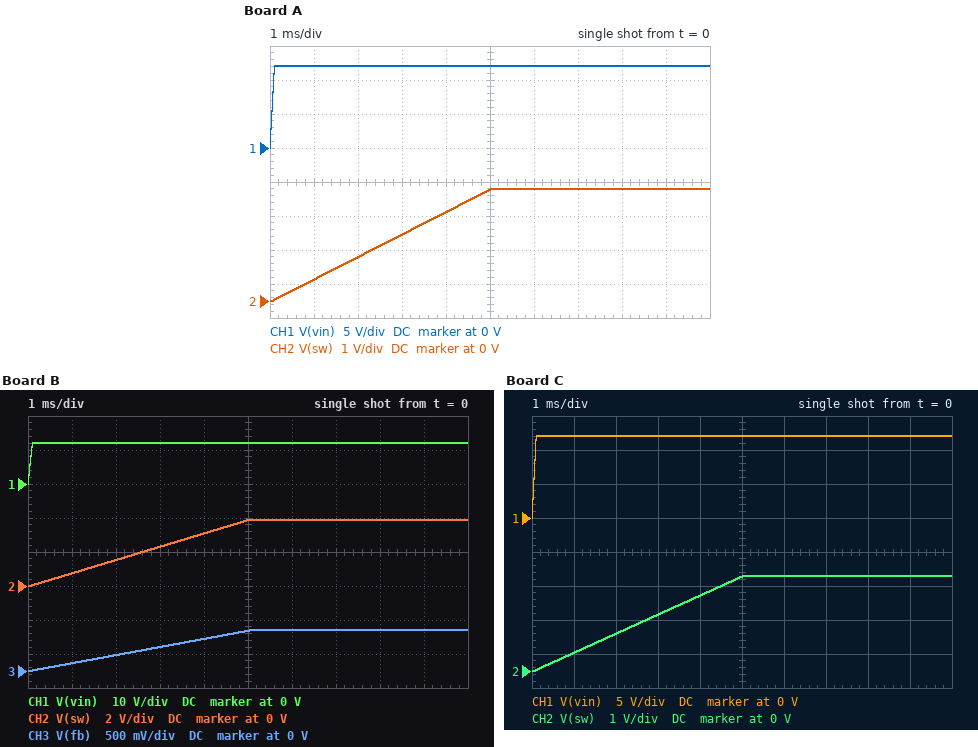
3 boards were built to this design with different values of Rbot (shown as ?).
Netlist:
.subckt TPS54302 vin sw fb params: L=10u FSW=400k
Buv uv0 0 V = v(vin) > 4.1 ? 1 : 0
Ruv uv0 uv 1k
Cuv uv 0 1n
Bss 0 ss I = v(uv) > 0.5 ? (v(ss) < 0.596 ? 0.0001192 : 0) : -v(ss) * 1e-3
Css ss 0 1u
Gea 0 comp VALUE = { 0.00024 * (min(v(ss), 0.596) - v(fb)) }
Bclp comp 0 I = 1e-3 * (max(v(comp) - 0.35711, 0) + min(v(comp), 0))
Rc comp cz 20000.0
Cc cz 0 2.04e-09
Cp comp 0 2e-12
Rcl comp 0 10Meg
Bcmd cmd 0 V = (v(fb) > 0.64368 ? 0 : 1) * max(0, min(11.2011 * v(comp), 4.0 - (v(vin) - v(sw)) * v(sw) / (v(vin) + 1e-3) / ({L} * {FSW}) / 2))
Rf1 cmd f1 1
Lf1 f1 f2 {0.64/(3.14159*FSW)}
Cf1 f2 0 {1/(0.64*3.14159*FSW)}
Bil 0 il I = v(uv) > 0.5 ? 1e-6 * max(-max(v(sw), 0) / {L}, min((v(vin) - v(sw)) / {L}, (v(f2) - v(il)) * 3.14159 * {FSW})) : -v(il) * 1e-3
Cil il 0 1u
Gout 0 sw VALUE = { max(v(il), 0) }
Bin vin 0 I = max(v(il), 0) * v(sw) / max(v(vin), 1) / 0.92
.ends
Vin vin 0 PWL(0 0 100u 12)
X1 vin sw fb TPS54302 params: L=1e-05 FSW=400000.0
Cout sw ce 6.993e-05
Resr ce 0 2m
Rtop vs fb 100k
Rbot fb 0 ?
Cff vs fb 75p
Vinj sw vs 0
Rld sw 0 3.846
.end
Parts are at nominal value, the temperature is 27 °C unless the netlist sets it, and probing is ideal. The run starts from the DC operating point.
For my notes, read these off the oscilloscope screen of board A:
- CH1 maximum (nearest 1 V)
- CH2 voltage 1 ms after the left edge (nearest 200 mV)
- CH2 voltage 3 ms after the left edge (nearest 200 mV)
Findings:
12 V
600 mV
2.0 V
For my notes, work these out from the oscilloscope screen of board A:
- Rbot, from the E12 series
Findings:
22 kΩ
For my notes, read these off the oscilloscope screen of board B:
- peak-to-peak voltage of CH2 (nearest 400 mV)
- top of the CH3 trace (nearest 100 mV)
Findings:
4.0 V
600 mV
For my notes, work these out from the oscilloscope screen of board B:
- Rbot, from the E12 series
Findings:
18 kΩ
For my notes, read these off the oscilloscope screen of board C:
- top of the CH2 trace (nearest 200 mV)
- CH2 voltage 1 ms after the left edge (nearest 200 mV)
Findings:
2.8 V
600 mV
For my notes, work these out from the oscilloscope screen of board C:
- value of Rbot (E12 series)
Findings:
27 kΩ
